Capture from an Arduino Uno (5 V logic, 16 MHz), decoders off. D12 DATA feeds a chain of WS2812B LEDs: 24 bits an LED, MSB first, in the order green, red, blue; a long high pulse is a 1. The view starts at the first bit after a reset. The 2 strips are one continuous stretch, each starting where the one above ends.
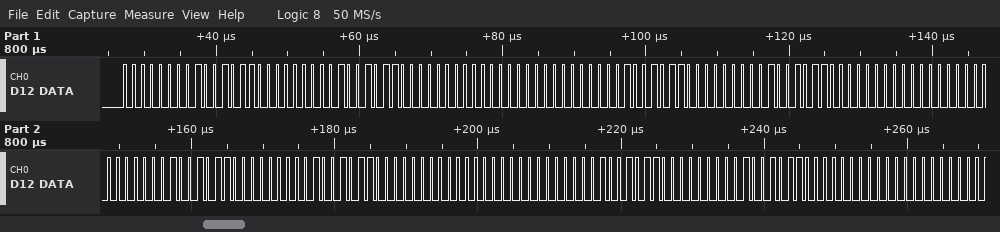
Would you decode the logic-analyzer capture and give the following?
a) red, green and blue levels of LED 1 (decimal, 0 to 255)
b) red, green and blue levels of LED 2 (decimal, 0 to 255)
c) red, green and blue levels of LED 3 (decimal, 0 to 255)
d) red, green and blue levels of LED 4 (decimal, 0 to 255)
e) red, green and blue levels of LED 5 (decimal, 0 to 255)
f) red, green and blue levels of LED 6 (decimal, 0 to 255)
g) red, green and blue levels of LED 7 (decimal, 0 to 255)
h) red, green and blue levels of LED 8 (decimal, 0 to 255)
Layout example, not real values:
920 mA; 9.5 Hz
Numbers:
150, 0, 0; 0, 150, 0; 150, 0, 0; 0, 150, 0; 150, 0, 0; 0, 150, 0; 150, 0, 0; 0, 150, 0
